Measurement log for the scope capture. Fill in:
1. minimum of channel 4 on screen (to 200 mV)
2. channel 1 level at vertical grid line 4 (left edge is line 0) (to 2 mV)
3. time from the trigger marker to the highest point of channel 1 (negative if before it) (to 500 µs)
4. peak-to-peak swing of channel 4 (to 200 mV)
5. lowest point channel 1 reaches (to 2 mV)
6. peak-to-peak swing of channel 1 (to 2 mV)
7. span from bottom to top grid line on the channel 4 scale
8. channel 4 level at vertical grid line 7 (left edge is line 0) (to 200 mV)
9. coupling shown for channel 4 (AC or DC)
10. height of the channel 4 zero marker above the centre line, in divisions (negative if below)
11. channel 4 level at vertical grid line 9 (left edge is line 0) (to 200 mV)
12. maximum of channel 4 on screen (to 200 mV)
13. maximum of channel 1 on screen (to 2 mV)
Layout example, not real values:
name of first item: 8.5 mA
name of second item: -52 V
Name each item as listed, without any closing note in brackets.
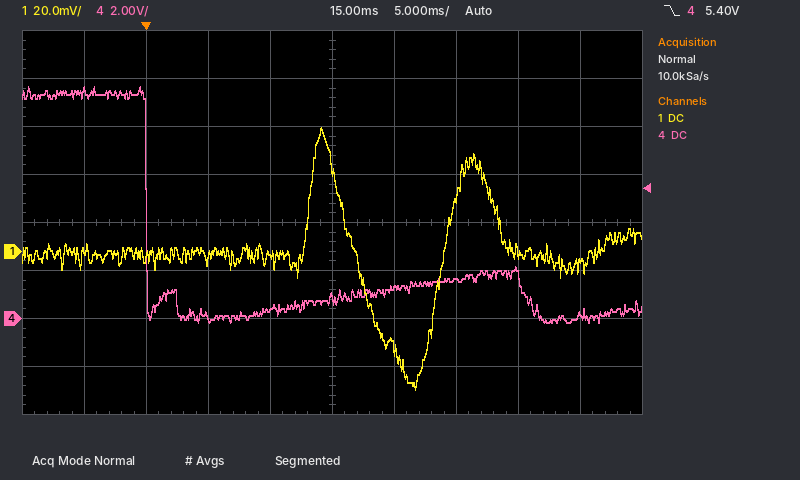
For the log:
minimum of channel 4 on screen: -200 mV
channel 1 level at vertical grid line 4 (left edge is line 0): -2 mV
time from the trigger marker to the highest point of channel 1 (negative if before it): +14.0 ms
peak-to-peak swing of channel 4: 9.8 V
lowest point channel 1 reaches: -58 mV
peak-to-peak swing of channel 1: 110 mV
span from bottom to top grid line on the channel 4 scale: 16 V
channel 4 level at vertical grid line 7 (left edge is line 0): 1.6 V
coupling shown for channel 4: DC
height of the channel 4 zero marker above the centre line, in divisions: -2.0 div
channel 4 level at vertical grid line 9 (left edge is line 0): 200 mV
maximum of channel 4 on screen: 9.6 V
maximum of channel 1 on screen: 52 mV
